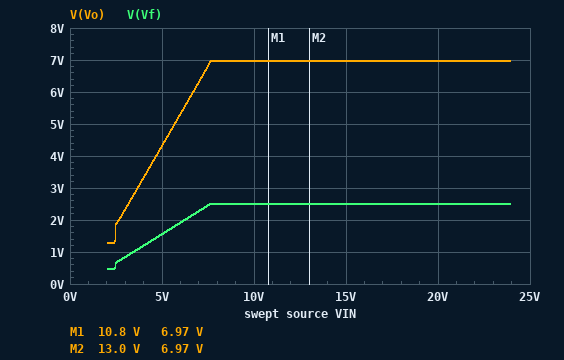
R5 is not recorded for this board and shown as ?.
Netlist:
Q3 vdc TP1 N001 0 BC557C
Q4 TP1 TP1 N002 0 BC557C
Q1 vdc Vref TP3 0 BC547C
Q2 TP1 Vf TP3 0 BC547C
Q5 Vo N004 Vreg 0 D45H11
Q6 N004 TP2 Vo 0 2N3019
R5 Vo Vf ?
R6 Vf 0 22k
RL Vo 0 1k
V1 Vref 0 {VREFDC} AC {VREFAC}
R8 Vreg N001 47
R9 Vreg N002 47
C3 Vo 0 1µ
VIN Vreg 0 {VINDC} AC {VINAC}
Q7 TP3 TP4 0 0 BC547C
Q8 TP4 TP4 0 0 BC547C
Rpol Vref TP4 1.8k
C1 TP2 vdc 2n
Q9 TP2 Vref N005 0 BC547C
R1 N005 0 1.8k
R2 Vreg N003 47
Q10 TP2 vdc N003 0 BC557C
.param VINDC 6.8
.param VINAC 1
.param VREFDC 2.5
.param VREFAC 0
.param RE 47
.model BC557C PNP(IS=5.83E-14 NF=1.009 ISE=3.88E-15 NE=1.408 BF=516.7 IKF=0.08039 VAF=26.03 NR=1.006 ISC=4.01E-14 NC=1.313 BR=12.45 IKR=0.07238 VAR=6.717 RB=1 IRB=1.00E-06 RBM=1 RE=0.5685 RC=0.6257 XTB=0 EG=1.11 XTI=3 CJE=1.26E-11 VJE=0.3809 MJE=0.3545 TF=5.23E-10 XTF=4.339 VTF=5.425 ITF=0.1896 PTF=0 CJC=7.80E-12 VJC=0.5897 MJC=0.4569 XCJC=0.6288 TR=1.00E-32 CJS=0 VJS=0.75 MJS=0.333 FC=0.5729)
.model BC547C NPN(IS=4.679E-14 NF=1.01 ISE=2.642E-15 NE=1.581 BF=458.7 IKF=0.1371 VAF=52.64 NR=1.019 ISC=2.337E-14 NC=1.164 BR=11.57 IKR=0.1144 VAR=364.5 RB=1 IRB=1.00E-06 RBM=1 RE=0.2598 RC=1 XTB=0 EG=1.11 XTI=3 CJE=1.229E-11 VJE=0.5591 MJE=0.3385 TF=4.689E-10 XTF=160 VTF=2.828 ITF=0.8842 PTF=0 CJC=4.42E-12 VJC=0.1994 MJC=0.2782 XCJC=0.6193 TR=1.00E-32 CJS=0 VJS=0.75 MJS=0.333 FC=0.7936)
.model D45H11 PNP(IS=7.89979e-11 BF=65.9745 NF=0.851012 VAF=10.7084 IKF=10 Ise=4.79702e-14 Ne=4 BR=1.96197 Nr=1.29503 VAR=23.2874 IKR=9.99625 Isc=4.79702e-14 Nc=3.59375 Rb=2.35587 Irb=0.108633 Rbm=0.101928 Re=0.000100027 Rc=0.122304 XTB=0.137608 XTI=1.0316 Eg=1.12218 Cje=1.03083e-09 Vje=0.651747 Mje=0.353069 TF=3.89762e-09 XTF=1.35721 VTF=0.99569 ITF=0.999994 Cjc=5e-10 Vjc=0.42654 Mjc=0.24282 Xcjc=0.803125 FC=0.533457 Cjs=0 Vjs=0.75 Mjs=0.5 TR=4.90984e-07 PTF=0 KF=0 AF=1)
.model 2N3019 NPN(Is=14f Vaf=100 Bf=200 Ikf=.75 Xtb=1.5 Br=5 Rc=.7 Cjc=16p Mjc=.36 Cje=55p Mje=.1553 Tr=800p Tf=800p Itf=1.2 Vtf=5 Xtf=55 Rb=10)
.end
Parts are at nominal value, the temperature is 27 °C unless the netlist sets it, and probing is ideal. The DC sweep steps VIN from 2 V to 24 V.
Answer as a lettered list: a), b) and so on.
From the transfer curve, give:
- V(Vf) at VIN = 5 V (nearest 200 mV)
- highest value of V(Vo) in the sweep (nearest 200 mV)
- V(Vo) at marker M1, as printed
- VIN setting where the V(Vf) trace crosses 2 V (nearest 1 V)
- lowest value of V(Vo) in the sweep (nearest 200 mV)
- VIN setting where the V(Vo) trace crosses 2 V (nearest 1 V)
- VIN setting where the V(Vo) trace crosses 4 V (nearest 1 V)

a) 1.6 V
b) 7.0 V
c) 6.97 V
d) 6 V
e) 1.2 V
f) 3 V
g) 5 V
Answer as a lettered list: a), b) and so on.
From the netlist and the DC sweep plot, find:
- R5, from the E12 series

a) 39 kΩ
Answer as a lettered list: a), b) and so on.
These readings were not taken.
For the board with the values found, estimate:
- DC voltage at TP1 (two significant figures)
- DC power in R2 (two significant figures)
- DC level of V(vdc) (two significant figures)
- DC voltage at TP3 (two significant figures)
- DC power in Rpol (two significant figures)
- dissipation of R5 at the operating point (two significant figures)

a) 6.5 V
b) 210 µW
c) 6.0 V
d) 1.9 V
e) 2.0 mW
f) 390 µW
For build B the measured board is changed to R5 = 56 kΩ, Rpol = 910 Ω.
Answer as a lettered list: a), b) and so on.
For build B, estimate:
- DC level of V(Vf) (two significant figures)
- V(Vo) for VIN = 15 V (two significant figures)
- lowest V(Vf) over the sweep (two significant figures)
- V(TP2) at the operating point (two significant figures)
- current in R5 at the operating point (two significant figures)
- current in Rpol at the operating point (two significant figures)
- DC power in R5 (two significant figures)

a) 1.7 V
b) 9.0 V
c) 360 mV
d) 6.6 V
e) 78 µA
f) 2.0 mA
g) 340 µW
